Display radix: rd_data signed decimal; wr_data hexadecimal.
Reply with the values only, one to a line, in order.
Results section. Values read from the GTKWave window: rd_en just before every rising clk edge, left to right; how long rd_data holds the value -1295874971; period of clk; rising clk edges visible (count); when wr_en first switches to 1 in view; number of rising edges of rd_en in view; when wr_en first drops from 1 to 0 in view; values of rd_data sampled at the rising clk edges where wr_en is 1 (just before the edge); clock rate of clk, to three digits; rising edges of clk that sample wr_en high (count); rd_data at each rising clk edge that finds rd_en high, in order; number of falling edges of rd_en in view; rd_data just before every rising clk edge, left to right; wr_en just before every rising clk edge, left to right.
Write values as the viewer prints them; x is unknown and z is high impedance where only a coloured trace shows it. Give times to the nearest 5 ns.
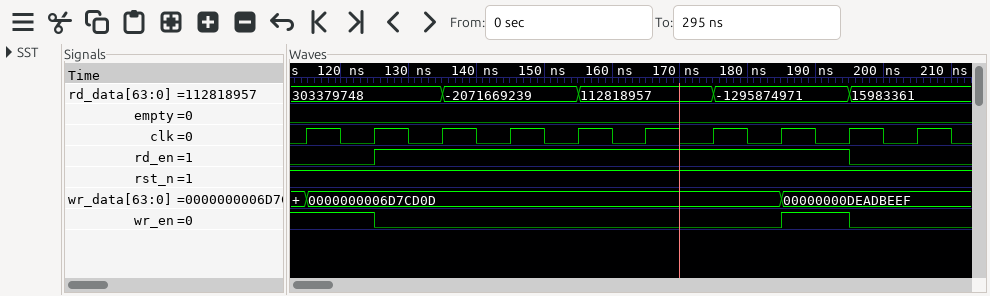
0 0 1 1 1 1 1 1 1 0
20 ns
10 ns
10
185 ns
1
125 ns
303379748, 303379748, -1295874971
100 MHz
3
303379748, -2071669239, -2071669239, 112818957, 112818957, -1295874971, -1295874971
1
303379748, 303379748, 303379748, -2071669239, -2071669239, 112818957, 112818957, -1295874971, -1295874971, 15983361
1 1 0 0 0 0 0 0 1 0
